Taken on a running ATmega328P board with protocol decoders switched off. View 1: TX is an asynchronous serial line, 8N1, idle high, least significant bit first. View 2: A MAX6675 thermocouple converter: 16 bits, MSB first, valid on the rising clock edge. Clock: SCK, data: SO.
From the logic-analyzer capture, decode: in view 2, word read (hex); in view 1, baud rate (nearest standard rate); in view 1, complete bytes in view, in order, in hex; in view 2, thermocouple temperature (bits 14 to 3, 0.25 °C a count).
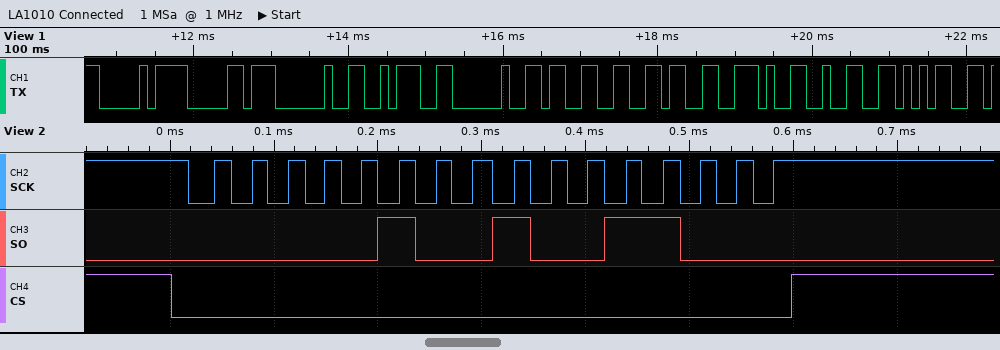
0x0498
9600 baud
0xD0 0xB0 0x20 0x3A 0x20 0x33 0x36 0x2E 0x32 0x35
36.75 °C
